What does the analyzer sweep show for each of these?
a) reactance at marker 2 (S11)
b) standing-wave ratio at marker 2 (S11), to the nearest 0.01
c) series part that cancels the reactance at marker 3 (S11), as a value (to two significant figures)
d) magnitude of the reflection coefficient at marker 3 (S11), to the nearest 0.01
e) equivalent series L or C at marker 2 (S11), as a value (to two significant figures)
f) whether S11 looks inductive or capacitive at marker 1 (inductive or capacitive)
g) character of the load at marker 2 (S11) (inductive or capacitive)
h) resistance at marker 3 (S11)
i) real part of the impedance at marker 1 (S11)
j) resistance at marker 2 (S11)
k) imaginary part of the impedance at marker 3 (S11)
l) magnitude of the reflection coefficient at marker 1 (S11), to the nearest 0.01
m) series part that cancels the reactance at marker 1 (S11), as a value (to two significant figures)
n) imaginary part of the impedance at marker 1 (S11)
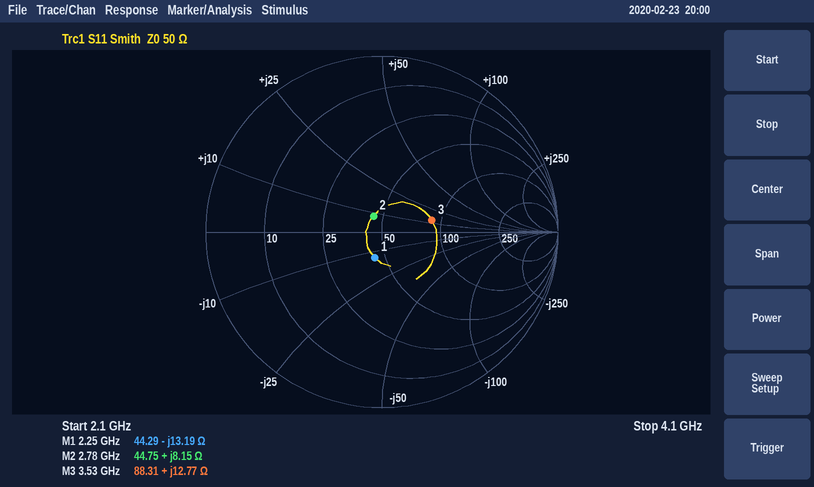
+8.15 Ω
1.23
3.5 pF
0.29
470 pH
capacitive
inductive
88.31 Ω
44.29 Ω
44.75 Ω
+12.77 Ω
0.15
930 pH
-13.19 Ω
